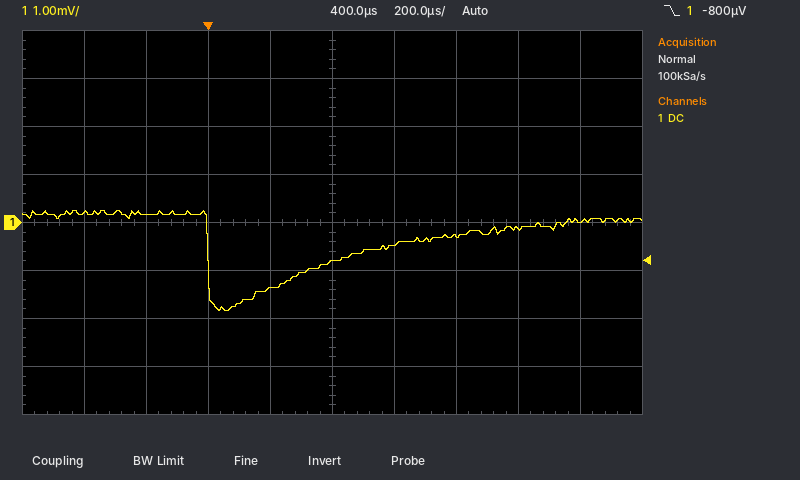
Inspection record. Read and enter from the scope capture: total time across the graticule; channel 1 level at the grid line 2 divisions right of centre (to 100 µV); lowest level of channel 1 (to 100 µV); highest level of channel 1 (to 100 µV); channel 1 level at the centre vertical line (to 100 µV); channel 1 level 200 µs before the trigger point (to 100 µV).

2 ms
-300 µV
-1.8 mV
200 µV
-800 µV
200 µV
